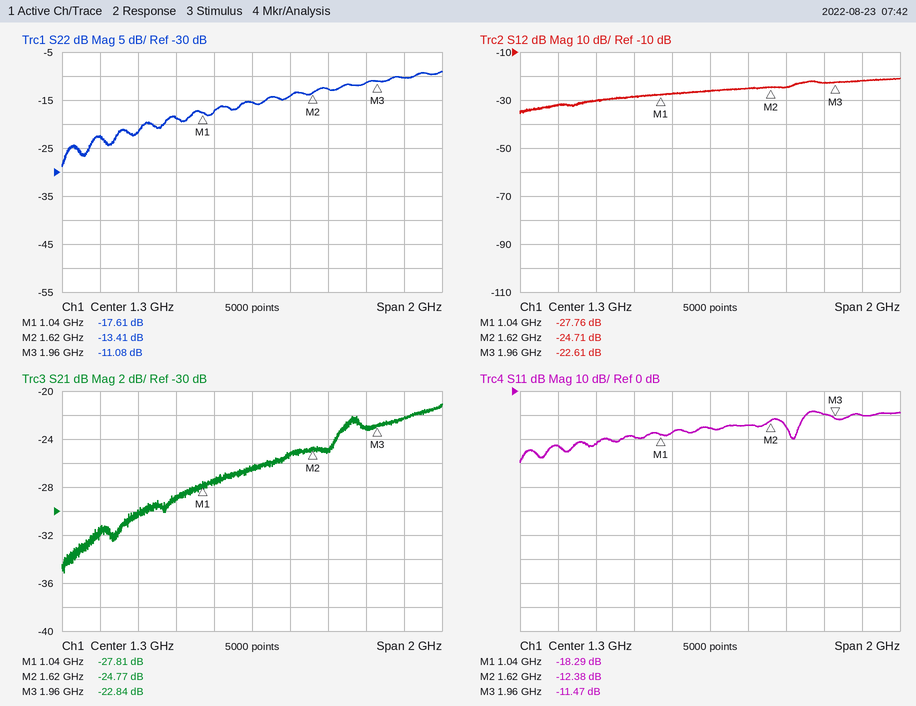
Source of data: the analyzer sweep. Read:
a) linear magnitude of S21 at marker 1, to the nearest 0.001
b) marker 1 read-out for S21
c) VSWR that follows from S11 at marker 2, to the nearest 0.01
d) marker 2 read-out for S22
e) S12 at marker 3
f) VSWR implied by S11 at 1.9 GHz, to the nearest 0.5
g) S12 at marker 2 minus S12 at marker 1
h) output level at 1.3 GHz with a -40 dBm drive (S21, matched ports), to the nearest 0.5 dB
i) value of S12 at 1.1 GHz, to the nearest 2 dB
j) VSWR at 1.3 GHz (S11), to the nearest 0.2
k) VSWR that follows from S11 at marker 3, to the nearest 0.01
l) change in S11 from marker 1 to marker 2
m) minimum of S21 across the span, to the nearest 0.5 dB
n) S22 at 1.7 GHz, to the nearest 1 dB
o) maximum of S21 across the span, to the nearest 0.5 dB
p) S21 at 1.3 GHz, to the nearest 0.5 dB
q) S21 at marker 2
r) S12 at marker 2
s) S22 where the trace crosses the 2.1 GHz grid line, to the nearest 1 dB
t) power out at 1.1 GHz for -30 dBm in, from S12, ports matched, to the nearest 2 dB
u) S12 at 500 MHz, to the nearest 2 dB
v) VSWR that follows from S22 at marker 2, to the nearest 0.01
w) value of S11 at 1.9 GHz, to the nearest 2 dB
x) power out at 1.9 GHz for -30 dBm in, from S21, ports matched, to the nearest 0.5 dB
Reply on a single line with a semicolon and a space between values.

0.041; -27.81 dB; 1.63; -13.41 dB; -22.61 dB; 2.0; 3.05 dB; -66.5 dBm; -28 dB; 1.4; 1.73; 5.91 dB; -35.0 dB; -13 dB; -21.0 dB; -26.5 dB; -24.77 dB; -24.71 dB; -10 dB; -58 dBm; -32 dB; 1.54; -10 dB; -53.0 dBm
